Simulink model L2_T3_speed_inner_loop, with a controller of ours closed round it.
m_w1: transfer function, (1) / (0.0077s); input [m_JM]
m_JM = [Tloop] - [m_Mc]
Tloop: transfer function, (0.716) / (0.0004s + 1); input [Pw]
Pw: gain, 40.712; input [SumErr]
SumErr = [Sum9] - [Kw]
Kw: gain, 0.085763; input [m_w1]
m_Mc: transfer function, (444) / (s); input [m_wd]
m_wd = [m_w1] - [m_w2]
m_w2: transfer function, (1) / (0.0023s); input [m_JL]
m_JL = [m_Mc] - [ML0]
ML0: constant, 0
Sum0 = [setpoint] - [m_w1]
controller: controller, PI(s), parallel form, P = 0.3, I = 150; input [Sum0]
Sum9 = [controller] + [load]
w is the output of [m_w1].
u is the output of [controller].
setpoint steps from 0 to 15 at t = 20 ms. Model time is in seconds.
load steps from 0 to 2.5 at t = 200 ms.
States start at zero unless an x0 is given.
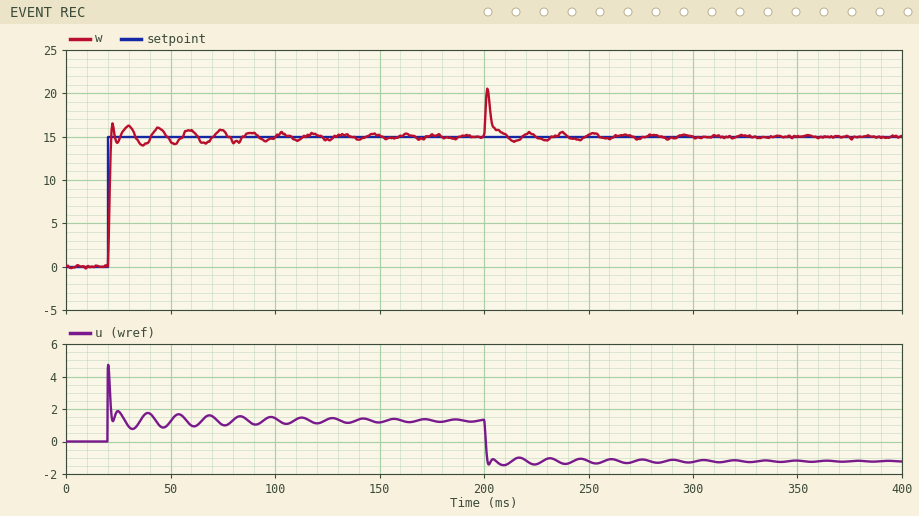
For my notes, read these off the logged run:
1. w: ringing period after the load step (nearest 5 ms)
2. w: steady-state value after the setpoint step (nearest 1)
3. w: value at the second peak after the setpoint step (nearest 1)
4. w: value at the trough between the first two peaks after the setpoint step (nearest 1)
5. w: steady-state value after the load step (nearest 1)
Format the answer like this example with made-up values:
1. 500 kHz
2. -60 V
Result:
1. 20 ms
2. 15
3. 16
4. 14
5. 15
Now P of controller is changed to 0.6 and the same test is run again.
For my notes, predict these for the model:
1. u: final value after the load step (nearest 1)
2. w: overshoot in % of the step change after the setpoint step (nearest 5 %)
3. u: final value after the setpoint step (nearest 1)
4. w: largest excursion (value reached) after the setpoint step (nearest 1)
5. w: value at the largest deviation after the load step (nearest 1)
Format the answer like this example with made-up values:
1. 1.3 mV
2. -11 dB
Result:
1. -1
2. 15 %
3. 1
4. 17
5. 19
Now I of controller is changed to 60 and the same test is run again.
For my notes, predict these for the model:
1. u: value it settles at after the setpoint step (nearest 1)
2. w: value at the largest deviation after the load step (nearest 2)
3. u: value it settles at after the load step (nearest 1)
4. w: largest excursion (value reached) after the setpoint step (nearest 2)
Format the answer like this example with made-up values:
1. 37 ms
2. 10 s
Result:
1. 1
2. 22
3. -1
4. 16
